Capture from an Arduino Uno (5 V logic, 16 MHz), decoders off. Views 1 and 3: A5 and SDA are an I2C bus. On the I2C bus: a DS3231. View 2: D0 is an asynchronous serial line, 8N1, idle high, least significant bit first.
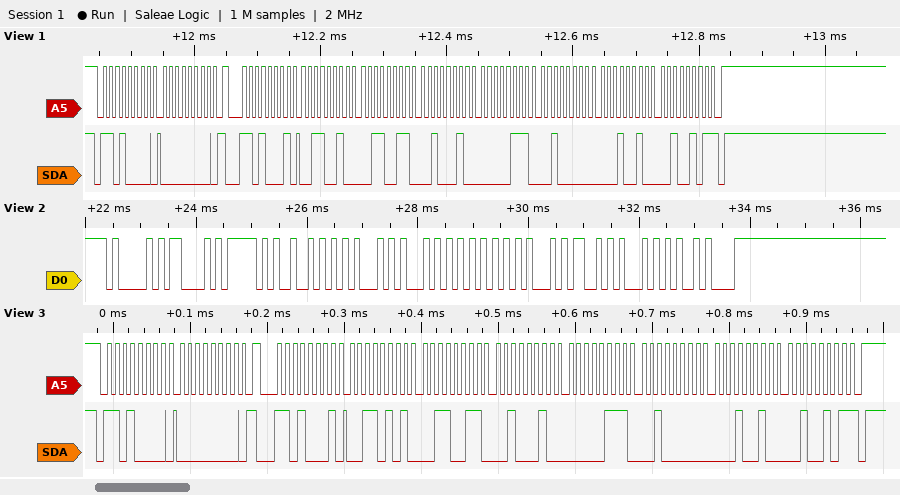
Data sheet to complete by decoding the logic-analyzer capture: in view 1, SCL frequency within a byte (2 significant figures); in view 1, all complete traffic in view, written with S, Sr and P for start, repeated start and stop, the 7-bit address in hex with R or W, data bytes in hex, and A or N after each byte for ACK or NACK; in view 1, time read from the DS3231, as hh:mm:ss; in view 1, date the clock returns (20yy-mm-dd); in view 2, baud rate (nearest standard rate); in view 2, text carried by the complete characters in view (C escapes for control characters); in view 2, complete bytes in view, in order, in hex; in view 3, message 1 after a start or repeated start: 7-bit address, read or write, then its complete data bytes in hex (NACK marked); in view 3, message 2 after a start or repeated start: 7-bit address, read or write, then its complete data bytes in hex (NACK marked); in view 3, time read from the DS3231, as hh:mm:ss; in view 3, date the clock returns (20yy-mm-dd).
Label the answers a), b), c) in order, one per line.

a) 100 kHz
b) S 68W A 00 A Sr 68R A 32 A 33 A 22 A 07 A 20 A 12 A 25 N P
c) 22:33:32
d) 2025-12-20
e) 9600 baud
f) "AC_REQUEST\n"
g) 41 43 5F 52 45 51 55 45 53 54 0A
h) 0x68 write: 00
i) 0x68 read: 35 33 22 07 20 12 25 NACK
j) 22:33:35
k) 2025-12-20
